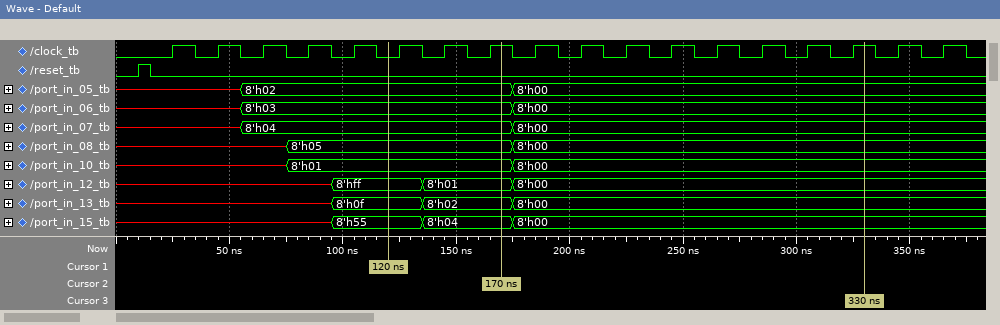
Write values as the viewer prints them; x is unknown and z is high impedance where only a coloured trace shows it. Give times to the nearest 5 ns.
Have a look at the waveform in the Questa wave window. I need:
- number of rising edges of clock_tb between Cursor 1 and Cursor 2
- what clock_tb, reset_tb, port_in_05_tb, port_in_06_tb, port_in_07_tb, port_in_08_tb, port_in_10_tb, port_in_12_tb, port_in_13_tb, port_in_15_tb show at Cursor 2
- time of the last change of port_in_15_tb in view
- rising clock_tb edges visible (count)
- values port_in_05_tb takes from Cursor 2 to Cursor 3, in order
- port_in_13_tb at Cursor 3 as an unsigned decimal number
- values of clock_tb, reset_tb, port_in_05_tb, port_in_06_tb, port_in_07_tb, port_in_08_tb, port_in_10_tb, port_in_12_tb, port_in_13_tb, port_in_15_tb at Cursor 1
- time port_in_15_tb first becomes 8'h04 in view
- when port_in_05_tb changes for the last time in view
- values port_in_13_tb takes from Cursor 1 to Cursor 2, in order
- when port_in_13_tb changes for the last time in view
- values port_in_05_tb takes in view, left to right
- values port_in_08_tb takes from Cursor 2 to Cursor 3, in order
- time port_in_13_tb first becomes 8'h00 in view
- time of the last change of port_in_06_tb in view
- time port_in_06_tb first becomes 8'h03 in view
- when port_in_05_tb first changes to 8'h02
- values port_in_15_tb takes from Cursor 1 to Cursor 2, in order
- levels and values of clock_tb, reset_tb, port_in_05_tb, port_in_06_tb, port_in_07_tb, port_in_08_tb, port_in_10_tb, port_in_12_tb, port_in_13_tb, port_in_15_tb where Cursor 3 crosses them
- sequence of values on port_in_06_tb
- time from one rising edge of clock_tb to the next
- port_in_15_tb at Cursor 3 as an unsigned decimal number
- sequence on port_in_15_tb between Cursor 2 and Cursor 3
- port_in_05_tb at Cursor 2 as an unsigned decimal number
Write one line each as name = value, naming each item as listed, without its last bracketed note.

number of rising edges of clock_tb between Cursor 1 and Cursor 2 = 3
what clock_tb, reset_tb, port_in_05_tb, port_in_06_tb, port_in_07_tb, port_in_08_tb, port_in_10_tb, port_in_12_tb, port_in_13_tb, port_in_15_tb show at Cursor 2 = clock_tb=1, reset_tb=0, port_in_05_tb=8'h02, port_in_06_tb=8'h03, port_in_07_tb=8'h04, port_in_08_tb=8'h05, port_in_10_tb=8'h01, port_in_12_tb=8'h01, port_in_13_tb=8'h02, port_in_15_tb=8'h04
time of the last change of port_in_15_tb in view = 175 ns
rising clock_tb edges visible = 18
values port_in_05_tb takes from Cursor 2 to Cursor 3, in order = 8'h02, 8'h00
port_in_13_tb at Cursor 3 as an unsigned decimal number = 0
values of clock_tb, reset_tb, port_in_05_tb, port_in_06_tb, port_in_07_tb, port_in_08_tb, port_in_10_tb, port_in_12_tb, port_in_13_tb, port_in_15_tb at Cursor 1 = clock_tb=0, reset_tb=0, port_in_05_tb=8'h02, port_in_06_tb=8'h03, port_in_07_tb=8'h04, port_in_08_tb=8'h05, port_in_10_tb=8'h01, port_in_12_tb=8'hff, port_in_13_tb=8'h0f, port_in_15_tb=8'h55
time port_in_15_tb first becomes 8'h04 in view = 135 ns
when port_in_05_tb changes for the last time in view = 175 ns
values port_in_13_tb takes from Cursor 1 to Cursor 2, in order = 8'h0f, 8'h02
when port_in_13_tb changes for the last time in view = 175 ns
values port_in_05_tb takes in view, left to right = x, 8'h02, 8'h00
values port_in_08_tb takes from Cursor 2 to Cursor 3, in order = 8'h05, 8'h00
time port_in_13_tb first becomes 8'h00 in view = 175 ns
time of the last change of port_in_06_tb in view = 175 ns
time port_in_06_tb first becomes 8'h03 in view = 55 ns
when port_in_05_tb first changes to 8'h02 = 55 ns
values port_in_15_tb takes from Cursor 1 to Cursor 2, in order = 8'h55, 8'h04
levels and values of clock_tb, reset_tb, port_in_05_tb, port_in_06_tb, port_in_07_tb, port_in_08_tb, port_in_10_tb, port_in_12_tb, port_in_13_tb, port_in_15_tb where Cursor 3 crosses them = clock_tb=1, reset_tb=0, port_in_05_tb=8'h00, port_in_06_tb=8'h00, port_in_07_tb=8'h00, port_in_08_tb=8'h00, port_in_10_tb=8'h00, port_in_12_tb=8'h00, port_in_13_tb=8'h00, port_in_15_tb=8'h00
sequence of values on port_in_06_tb = x, 8'h03, 8'h00
time from one rising edge of clock_tb to the next = 20 ns
port_in_15_tb at Cursor 3 as an unsigned decimal number = 0
sequence on port_in_15_tb between Cursor 2 and Cursor 3 = 8'h04, 8'h00
port_in_05_tb at Cursor 2 as an unsigned decimal number = 2
